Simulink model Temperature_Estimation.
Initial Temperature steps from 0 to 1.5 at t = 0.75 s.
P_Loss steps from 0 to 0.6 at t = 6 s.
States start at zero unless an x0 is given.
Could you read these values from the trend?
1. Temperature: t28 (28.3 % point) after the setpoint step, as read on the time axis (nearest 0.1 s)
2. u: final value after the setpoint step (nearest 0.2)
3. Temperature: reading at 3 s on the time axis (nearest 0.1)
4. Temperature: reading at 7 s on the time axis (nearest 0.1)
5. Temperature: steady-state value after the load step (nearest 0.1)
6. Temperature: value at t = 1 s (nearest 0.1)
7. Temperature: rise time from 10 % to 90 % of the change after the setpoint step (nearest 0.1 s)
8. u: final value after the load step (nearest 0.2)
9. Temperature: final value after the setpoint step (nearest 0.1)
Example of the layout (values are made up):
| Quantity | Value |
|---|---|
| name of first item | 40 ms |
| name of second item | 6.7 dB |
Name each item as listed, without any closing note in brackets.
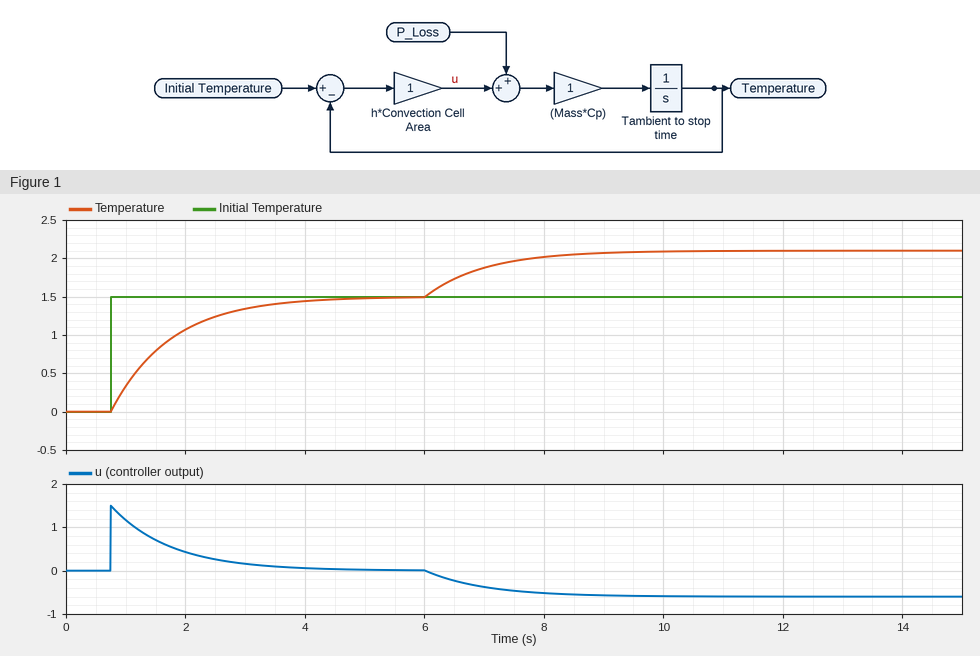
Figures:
| Quantity | Value |
|---|---|
| Temperature: t28 (28.3 % point) after the setpoint step, as read on the time axis | 1.1 s |
| u: final value after the setpoint step | 0.0 |
| Temperature: reading at 3 s on the time axis | 1.3 |
| Temperature: reading at 7 s on the time axis | 1.9 |
| Temperature: steady-state value after the load step | 2.1 |
| Temperature: value at t = 1 s | 0.3 |
| Temperature: rise time from 10 % to 90 % of the change after the setpoint step | 2.2 s |
| u: final value after the load step | -0.6 |
| Temperature: final value after the setpoint step | 1.5 |
